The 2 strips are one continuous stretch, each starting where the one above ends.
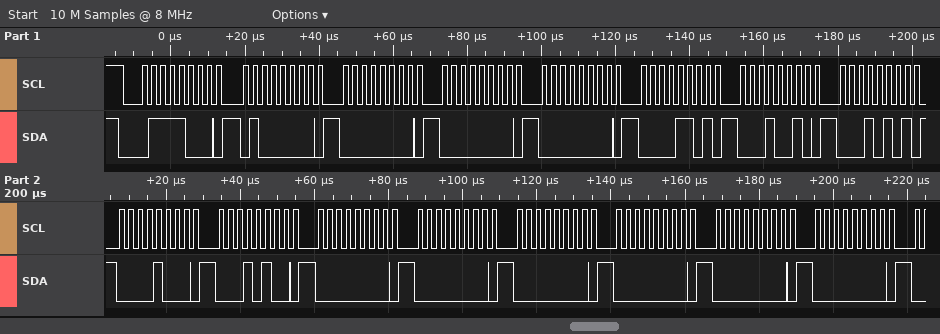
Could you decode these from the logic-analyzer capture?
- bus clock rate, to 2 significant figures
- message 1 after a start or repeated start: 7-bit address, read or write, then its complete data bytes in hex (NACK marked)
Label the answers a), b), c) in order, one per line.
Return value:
a) 400 kHz
b) 0x3C write: 40 00 00 00 0D 12 15 08 14 00 00 00 00 00 00
